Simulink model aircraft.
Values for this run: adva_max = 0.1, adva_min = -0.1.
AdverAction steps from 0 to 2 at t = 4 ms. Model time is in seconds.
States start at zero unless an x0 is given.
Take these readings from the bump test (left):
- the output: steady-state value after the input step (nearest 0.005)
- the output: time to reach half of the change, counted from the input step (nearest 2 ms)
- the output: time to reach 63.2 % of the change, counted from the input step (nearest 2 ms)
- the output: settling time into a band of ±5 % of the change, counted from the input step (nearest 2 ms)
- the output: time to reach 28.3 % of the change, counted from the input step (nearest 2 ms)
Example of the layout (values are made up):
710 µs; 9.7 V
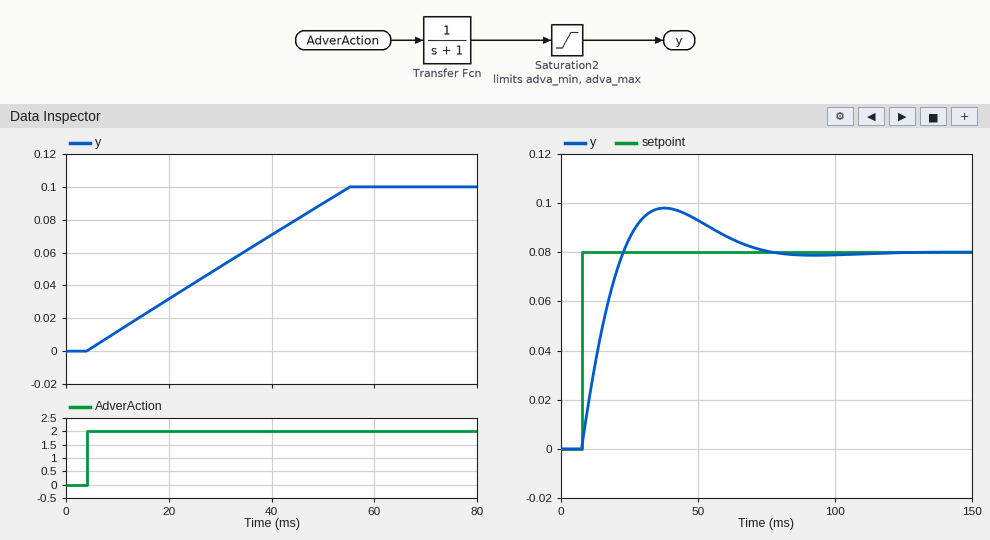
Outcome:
0.100; 26 ms; 32 ms; 48 ms; 14 ms
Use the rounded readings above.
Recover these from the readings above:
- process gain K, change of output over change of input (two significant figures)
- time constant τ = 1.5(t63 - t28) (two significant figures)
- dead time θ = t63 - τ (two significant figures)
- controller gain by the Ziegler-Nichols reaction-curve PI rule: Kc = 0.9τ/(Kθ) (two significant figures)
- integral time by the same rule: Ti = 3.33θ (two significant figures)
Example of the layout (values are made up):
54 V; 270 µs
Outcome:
0.050; 27 ms; 5.0 ms; 97; 17 ms
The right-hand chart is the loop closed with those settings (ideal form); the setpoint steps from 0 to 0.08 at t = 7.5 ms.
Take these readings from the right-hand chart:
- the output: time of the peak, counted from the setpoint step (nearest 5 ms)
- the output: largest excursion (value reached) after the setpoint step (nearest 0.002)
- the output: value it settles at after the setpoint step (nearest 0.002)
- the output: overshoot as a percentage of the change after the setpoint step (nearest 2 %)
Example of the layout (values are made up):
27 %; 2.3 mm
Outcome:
30 ms; 0.098; 0.080; 22 %
